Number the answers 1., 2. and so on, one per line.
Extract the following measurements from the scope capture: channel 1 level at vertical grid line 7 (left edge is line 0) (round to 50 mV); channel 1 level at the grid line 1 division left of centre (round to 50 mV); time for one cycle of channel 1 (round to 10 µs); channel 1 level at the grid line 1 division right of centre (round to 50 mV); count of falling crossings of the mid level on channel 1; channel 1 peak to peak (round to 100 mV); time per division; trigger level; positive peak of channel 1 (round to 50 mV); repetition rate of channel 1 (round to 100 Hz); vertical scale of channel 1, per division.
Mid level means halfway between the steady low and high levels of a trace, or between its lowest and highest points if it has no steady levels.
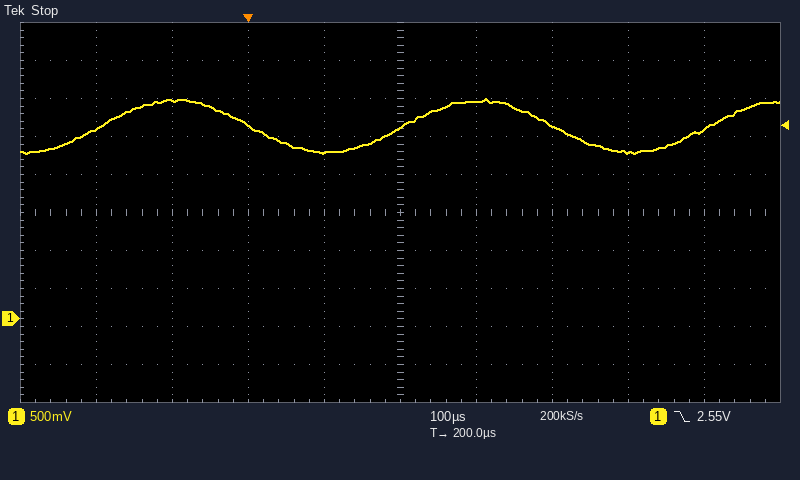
1. 2.55 V
2. 2.20 V
3. 400 µs
4. 2.85 V
5. 2
6. 700 mV
7. 100 µs
8. 2.55 V
9. 2.90 V
10. 2.5 kHz
11. 500 mV
